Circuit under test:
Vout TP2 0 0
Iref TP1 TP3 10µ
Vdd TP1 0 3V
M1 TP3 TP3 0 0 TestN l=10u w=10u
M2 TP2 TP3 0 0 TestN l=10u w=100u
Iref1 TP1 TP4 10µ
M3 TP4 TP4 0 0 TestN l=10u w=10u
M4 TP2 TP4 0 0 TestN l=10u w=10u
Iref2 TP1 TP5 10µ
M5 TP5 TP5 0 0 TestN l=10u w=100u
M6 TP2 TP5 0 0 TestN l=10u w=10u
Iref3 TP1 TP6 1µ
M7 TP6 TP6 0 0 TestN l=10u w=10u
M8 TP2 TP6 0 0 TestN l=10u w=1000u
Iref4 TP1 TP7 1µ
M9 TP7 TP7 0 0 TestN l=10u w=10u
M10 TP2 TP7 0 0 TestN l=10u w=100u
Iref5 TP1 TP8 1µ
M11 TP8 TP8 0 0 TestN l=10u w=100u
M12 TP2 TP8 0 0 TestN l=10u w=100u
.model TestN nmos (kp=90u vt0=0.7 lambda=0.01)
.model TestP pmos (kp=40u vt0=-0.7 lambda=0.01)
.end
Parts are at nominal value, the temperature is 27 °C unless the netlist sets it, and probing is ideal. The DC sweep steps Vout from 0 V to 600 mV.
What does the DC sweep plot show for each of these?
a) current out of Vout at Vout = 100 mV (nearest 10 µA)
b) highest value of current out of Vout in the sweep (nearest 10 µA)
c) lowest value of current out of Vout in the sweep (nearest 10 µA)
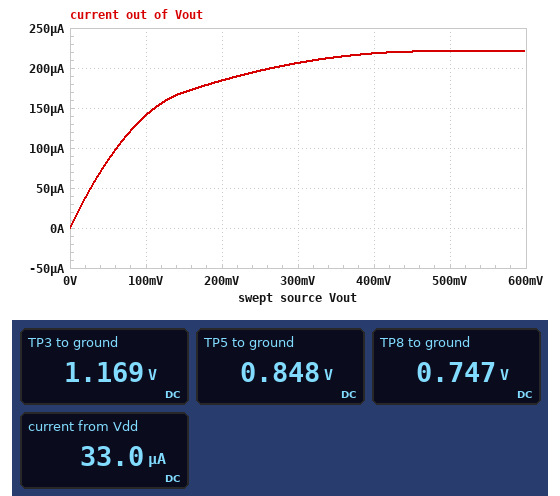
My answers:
140 µA
220 µA
0 A
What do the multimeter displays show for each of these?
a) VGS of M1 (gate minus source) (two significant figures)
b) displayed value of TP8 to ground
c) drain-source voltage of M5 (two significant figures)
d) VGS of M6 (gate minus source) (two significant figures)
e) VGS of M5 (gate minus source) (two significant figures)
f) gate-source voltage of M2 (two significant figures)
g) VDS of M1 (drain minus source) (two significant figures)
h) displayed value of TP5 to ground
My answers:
1.2 V
0.747 V
850 mV
850 mV
850 mV
1.2 V
1.2 V
0.848 V
